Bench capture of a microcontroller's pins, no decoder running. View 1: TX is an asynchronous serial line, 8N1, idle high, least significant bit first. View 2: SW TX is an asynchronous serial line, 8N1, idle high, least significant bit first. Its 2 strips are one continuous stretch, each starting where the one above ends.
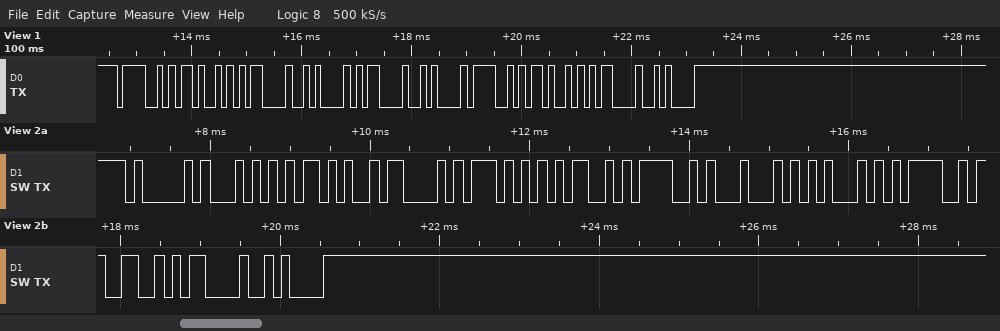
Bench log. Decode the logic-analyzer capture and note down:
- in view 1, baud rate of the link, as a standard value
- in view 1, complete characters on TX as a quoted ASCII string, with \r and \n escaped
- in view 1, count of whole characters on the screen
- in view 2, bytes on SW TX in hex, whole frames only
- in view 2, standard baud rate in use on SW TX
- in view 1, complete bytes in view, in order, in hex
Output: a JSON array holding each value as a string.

["9600 baud", "\"OK\\r\\n\\r\\nOK\\r\\n\"", "10", "0x41 0x54 0x2B 0x43 0x57 0x4D 0x4F 0x44 0x45 0x3D 0x33 0x0D 0x0A", "9600 baud", "0x4F 0x4B 0x0D 0x0A 0x0D 0x0A 0x4F 0x4B 0x0D 0x0A"]
